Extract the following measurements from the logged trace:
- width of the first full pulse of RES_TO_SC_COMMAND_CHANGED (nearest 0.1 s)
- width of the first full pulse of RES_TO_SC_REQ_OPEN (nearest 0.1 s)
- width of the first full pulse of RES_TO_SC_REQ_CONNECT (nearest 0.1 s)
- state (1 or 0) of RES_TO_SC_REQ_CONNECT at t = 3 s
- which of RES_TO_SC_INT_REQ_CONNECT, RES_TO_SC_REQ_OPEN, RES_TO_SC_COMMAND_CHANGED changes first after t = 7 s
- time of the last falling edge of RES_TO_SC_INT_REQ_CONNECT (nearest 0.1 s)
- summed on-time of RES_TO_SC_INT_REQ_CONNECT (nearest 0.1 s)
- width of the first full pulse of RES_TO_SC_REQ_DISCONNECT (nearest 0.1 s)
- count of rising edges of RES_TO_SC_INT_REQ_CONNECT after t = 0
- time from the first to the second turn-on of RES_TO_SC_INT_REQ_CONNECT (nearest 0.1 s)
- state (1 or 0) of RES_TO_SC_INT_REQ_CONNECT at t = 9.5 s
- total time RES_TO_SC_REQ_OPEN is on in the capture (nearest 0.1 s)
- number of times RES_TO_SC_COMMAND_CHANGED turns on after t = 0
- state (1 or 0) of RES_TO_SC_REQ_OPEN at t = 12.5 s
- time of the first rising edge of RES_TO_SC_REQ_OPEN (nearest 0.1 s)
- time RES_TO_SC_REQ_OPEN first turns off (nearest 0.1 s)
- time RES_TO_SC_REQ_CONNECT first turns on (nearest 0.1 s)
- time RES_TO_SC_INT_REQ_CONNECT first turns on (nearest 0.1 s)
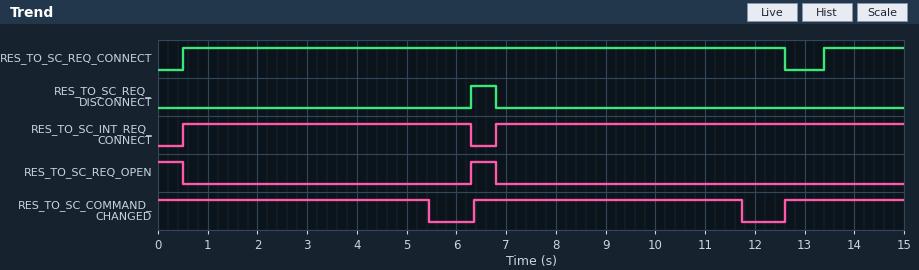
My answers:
5.4 s
0.5 s
12.1 s
1
RES_TO_SC_COMMAND_CHANGED
6.3 s
14.0 s
0.5 s
2
6.3 s
1
1.0 s
2
0
6.3 s
0.5 s
0.5 s
0.5 s
